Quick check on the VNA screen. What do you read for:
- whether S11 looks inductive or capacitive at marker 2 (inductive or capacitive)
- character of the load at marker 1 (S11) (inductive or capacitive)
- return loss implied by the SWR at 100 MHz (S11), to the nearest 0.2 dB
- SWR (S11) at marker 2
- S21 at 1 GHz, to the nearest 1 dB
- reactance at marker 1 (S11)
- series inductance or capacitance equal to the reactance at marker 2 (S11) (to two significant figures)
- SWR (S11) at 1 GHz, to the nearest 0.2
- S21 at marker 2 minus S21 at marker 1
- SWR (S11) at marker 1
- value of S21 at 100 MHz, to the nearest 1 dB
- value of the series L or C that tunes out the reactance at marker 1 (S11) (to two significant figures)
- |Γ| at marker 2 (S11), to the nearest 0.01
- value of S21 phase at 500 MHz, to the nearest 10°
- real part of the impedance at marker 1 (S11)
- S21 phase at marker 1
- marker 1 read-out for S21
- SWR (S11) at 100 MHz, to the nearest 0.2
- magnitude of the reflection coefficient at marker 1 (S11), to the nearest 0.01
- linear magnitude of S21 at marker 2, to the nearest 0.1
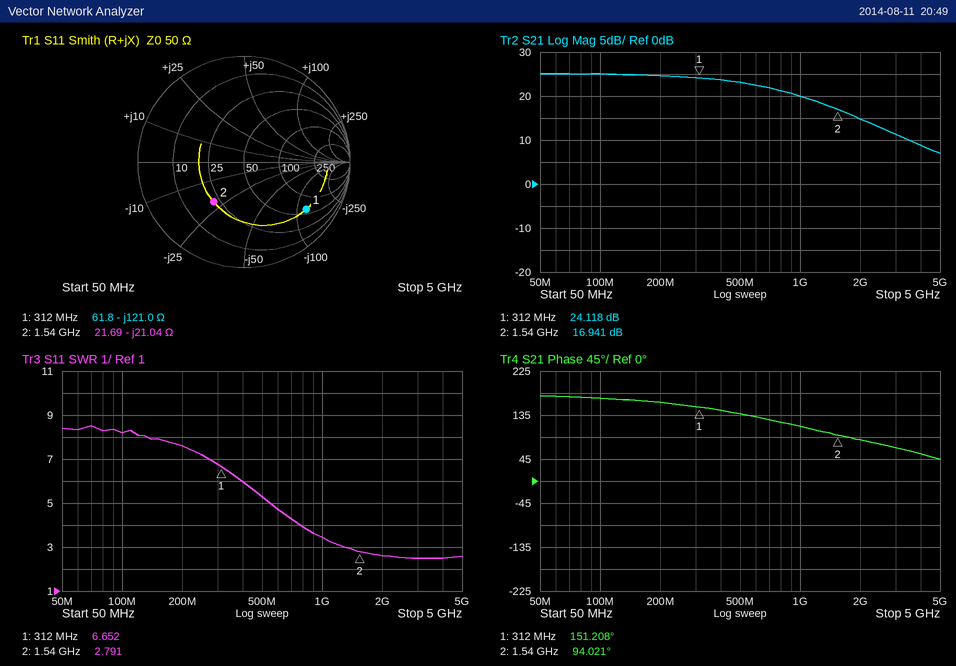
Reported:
capacitive
capacitive
2.2 dB
2.791
20 dB
-121.0 Ω
4.9 pF
3.4
-7.177 dB
6.652
25 dB
62 nH
0.47
140°
61.8 Ω
151.208°
24.118 dB
8.2
0.74
7.0
